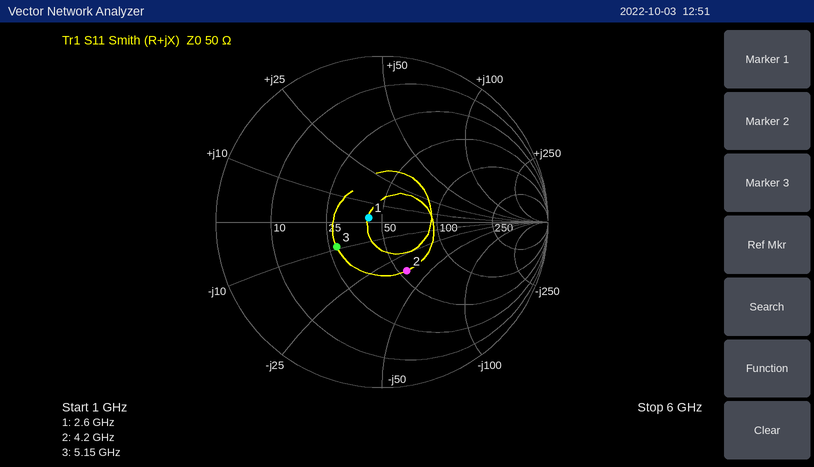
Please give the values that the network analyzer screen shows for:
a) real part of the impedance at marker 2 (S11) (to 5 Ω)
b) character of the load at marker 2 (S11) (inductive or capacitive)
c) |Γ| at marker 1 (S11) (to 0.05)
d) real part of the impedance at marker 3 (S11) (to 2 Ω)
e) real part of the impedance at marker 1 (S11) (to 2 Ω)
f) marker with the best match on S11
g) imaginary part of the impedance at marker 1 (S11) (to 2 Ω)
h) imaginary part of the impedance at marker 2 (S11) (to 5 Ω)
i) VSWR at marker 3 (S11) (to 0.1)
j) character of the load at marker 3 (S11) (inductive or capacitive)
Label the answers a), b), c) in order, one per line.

a) 55 Ω
b) capacitive
c) 0.10
d) 28 Ω
e) 42 Ω
f) marker 1
g) +2 Ω
h) -35 Ω
i) 1.9
j) capacitive
